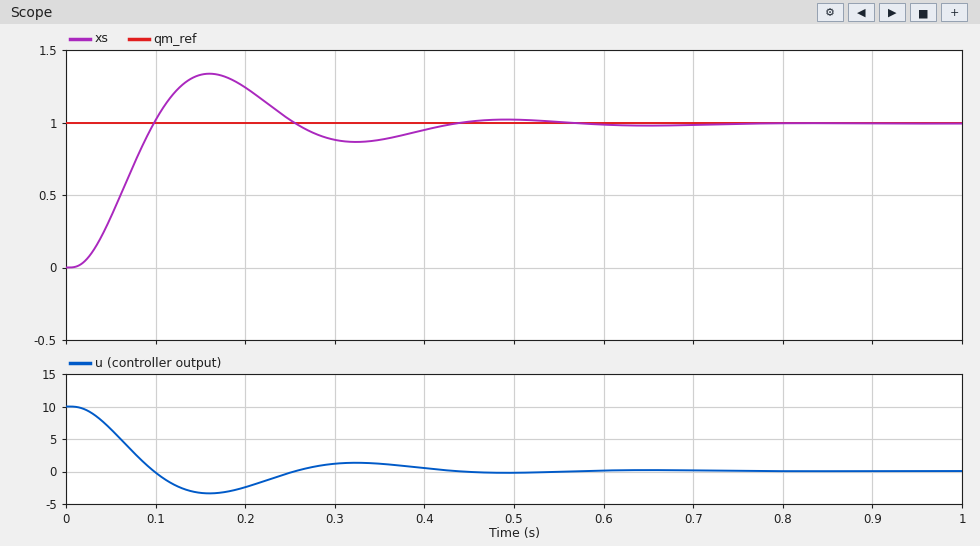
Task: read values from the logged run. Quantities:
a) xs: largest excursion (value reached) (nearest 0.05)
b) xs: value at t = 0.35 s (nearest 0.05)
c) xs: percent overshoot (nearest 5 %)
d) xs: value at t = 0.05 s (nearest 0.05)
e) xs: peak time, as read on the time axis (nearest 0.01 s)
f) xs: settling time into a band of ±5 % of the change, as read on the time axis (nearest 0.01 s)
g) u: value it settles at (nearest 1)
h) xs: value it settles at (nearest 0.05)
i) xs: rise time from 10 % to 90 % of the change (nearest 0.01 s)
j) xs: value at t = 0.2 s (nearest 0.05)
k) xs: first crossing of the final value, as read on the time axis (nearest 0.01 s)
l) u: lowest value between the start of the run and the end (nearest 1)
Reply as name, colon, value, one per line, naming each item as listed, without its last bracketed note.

xs: largest excursion (value reached): 1.35
xs: value at t = 0.35 s: 0.90
xs: percent overshoot: 35 %
xs: value at t = 0.05 s: 0.35
xs: peak time, as read on the time axis: 0.16 s
xs: settling time into a band of ±5 % of the change, as read on the time axis: 0.40 s
u: value it settles at: 0
xs: value it settles at: 1.00
xs: rise time from 10 % to 90 % of the change: 0.06 s
xs: value at t = 0.2 s: 1.25
xs: first crossing of the final value, as read on the time axis: 0.10 s
u: lowest value between the start of the run and the end: -3
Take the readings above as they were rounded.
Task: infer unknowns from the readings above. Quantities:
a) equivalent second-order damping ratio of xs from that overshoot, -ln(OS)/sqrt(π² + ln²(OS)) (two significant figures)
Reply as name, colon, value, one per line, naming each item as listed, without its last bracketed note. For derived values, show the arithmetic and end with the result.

equivalent second-order damping ratio of xs from that overshoot, -ln(OS)/sqrt(π² + ln²(OS)): ln(0.35) = -1.050; 1.050 / sqrt(9.870 + 1.102) = 0.32
